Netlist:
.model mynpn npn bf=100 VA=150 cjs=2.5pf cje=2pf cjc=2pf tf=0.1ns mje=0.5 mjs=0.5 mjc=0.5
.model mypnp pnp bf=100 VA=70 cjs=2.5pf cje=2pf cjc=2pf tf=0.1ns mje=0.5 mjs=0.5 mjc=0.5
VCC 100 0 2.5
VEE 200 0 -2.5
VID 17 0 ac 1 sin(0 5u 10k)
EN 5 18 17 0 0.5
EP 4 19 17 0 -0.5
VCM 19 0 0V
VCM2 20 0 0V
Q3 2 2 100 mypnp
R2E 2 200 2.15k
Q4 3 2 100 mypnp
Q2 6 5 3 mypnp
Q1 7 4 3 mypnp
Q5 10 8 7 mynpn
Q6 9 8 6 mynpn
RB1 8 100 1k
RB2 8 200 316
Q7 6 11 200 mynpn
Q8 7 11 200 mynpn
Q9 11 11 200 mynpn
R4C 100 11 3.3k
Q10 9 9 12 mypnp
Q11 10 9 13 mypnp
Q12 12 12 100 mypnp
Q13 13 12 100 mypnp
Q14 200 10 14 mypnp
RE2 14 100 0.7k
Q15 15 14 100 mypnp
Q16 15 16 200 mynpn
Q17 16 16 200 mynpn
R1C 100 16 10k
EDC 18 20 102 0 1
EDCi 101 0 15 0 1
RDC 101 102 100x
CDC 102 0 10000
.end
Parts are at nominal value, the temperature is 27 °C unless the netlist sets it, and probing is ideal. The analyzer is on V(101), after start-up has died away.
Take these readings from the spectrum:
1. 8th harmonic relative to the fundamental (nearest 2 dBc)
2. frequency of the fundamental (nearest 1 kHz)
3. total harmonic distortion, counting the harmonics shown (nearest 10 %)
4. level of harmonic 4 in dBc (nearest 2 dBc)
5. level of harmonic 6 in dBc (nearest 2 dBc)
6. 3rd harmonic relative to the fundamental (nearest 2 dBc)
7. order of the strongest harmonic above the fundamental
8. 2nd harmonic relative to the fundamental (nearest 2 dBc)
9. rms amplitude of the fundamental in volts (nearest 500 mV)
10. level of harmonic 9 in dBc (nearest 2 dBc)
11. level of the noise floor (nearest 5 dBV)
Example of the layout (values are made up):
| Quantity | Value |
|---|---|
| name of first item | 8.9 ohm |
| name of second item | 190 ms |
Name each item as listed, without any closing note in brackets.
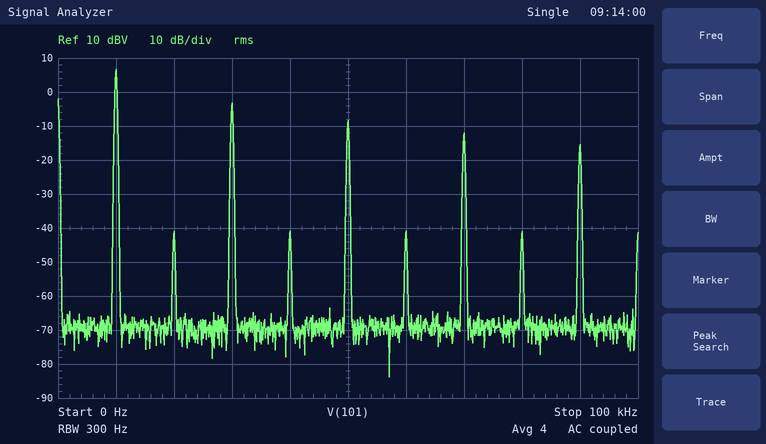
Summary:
| Quantity | Value |
|---|---|
| 8th harmonic relative to the fundamental | -48 dBc |
| frequency of the fundamental | 10 kHz |
| total harmonic distortion, counting the harmonics shown | 40 % |
| level of harmonic 4 in dBc | -48 dBc |
| level of harmonic 6 in dBc | -48 dBc |
| 3rd harmonic relative to the fundamental | -10 dBc |
| order of the strongest harmonic above the fundamental | 3 |
| 2nd harmonic relative to the fundamental | -48 dBc |
| rms amplitude of the fundamental in volts | 2.0 V |
| level of harmonic 9 in dBc | -22 dBc |
| level of the noise floor | -70 dBV |
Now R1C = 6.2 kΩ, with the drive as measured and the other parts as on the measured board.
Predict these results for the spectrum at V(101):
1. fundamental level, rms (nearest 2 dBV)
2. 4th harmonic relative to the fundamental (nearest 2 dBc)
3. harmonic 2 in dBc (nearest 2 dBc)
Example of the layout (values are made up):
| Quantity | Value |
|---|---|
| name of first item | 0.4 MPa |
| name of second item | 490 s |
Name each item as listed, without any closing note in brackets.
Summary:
| Quantity | Value |
|---|---|
| fundamental level, rms | 6 dBV |
| 4th harmonic relative to the fundamental | -46 dBc |
| harmonic 2 in dBc | -46 dBc |
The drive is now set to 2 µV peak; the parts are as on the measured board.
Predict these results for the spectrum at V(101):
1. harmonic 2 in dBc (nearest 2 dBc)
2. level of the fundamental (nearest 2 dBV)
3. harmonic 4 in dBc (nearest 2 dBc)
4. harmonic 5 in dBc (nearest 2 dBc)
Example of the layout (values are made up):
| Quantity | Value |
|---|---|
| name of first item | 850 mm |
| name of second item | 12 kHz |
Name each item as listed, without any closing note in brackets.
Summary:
| Quantity | Value |
|---|---|
| harmonic 2 in dBc | -44 dBc |
| level of the fundamental | 6 dBV |
| harmonic 4 in dBc | -44 dBc |
| harmonic 5 in dBc | -18 dBc |
